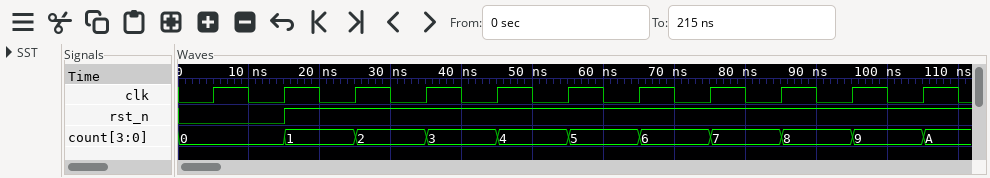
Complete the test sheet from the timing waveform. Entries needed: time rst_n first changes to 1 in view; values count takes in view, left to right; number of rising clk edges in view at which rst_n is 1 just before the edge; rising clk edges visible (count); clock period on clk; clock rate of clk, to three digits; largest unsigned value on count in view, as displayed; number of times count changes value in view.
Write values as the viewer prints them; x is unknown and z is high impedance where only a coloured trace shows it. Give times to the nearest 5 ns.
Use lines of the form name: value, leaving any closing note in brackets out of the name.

time rst_n first changes to 1 in view: 15 ns
values count takes in view, left to right: 0, 1, 2, 3, 4, 5, 6, 7, 8, 9, A
number of rising clk edges in view at which rst_n is 1 just before the edge: 9
rising clk edges visible: 11
clock period on clk: 10 ns
clock rate of clk, to three digits: 100 MHz
largest unsigned value on count in view, as displayed: A
number of times count changes value in view: 10
